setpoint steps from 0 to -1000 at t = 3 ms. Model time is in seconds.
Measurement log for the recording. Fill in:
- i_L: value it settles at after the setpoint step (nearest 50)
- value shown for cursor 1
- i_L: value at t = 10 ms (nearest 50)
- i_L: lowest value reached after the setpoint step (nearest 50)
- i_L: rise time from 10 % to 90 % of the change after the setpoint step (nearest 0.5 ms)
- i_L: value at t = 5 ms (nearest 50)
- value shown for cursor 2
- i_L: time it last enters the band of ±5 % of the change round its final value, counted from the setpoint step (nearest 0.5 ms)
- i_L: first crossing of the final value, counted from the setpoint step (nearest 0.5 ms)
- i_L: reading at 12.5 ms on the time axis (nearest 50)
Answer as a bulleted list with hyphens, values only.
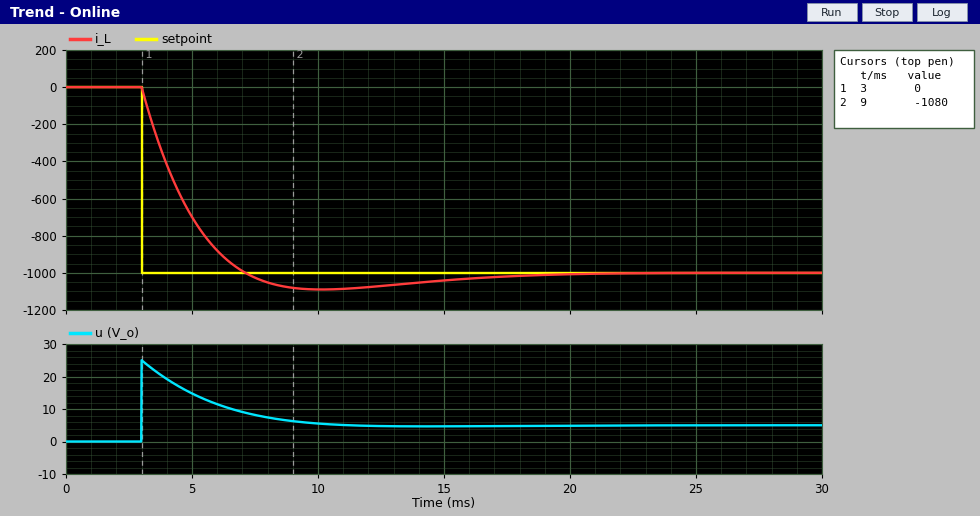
- -1000
- 0
- -1100
- -1100
- 3.0 ms
- -700
- -1080
- 11.0 ms
- 4.0 ms
- -1050
